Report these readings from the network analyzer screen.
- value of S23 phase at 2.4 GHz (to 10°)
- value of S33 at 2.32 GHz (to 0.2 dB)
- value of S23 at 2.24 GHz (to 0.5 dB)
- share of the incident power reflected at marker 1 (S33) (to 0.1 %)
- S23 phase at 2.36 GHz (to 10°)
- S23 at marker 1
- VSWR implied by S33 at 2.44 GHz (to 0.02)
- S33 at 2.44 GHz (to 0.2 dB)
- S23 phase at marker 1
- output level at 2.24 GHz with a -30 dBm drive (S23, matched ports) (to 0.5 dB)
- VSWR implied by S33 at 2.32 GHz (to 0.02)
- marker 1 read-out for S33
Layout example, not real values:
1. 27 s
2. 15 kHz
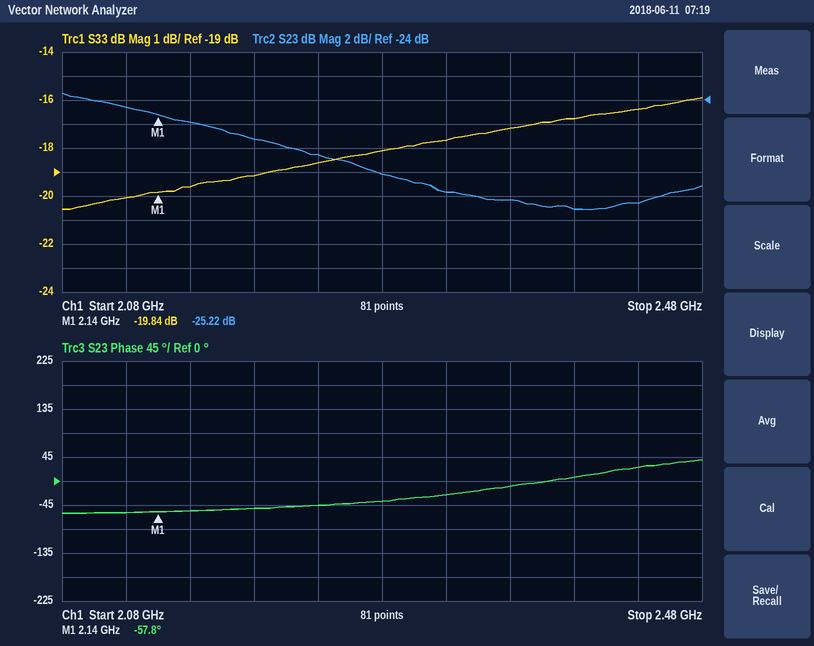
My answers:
1. 10°
2. -17.6 dB
3. -28.5 dB
4. 1.0 %
5. -10°
6. -25.22 dB
7. 1.36
8. -16.4 dB
9. -57.8°
10. -58.5 dBm
11. 1.30
12. -19.84 dB
